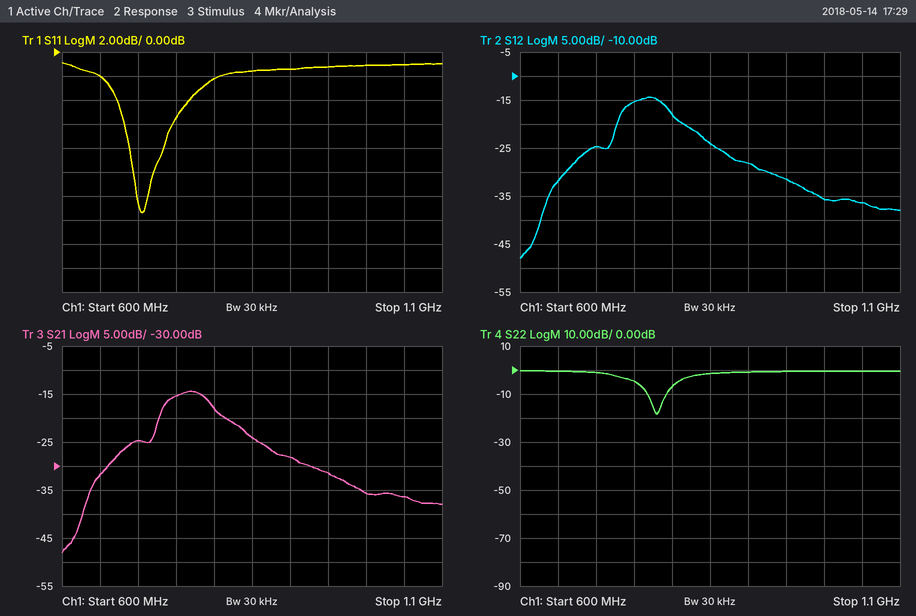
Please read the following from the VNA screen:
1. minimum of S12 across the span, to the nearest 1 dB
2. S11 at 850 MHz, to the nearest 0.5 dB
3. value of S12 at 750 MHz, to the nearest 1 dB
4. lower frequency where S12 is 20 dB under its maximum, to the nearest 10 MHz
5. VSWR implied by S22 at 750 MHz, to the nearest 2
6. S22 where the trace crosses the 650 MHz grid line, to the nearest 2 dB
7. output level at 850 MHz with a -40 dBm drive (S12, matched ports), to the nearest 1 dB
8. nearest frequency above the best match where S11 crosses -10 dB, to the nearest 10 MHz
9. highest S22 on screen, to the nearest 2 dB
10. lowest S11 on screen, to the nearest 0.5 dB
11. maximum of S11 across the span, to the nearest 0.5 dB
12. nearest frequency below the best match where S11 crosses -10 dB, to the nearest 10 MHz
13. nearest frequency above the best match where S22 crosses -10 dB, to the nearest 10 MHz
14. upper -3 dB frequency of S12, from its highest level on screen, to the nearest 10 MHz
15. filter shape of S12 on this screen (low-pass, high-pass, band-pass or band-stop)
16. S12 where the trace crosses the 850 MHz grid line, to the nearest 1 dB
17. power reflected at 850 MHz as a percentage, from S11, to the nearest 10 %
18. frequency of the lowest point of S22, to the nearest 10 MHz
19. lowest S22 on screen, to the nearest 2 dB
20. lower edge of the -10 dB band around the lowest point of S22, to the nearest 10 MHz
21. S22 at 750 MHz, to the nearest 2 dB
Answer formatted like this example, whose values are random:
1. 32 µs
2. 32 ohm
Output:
1. -48 dB
2. -1.5 dB
3. -15 dB
4. 640 MHz
5. 4
6. 0 dB
7. -64 dBm
8. 720 MHz
9. 0 dB
10. -13.5 dB
11. -1.0 dB
12. 690 MHz
13. 790 MHz
14. 800 MHz
15. band-pass
16. -24 dB
17. 70 %
18. 780 MHz
19. -18 dB
20. 770 MHz
21. -4 dB
